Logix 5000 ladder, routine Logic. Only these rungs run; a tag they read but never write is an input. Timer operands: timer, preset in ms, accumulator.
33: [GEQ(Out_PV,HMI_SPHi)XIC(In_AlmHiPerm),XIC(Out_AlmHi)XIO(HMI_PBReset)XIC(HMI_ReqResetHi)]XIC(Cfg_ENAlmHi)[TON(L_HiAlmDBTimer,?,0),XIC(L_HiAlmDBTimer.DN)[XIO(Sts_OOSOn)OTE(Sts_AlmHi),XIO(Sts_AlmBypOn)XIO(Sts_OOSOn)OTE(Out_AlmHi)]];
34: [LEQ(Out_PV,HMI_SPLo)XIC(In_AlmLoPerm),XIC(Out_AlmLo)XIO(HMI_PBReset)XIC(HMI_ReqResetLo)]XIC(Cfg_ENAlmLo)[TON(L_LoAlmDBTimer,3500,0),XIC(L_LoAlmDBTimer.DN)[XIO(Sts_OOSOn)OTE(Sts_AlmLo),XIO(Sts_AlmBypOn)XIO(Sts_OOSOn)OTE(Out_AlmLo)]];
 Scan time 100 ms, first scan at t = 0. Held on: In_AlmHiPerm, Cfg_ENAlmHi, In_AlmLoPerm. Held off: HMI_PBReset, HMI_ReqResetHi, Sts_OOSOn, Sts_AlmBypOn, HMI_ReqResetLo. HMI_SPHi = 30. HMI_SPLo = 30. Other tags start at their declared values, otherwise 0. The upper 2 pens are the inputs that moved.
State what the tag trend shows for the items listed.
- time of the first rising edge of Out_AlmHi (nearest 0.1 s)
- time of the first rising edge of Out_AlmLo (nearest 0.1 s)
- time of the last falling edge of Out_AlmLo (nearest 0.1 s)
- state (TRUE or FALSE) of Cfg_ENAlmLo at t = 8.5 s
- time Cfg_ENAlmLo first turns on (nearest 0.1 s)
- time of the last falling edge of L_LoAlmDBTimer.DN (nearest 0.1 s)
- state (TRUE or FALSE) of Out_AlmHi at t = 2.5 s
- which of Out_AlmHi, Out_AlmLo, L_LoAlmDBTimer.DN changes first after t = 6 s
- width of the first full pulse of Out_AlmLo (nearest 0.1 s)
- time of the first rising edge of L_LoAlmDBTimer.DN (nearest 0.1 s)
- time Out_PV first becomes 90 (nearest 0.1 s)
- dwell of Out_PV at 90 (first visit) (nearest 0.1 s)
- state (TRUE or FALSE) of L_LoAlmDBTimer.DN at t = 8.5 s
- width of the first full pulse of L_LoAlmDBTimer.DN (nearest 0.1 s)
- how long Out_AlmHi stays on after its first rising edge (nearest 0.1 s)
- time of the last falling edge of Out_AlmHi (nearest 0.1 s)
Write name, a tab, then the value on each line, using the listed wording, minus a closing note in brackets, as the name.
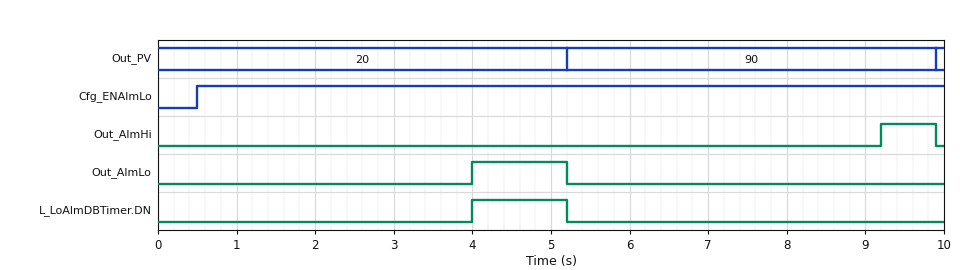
time of the first rising edge of Out_AlmHi	9.2 s
time of the first rising edge of Out_AlmLo	4.0 s
time of the last falling edge of Out_AlmLo	5.2 s
state (TRUE or FALSE) of Cfg_ENAlmLo at t = 8.5 s	TRUE
time Cfg_ENAlmLo first turns on	0.5 s
time of the last falling edge of L_LoAlmDBTimer.DN	5.2 s
state (TRUE or FALSE) of Out_AlmHi at t = 2.5 s	FALSE
which of Out_AlmHi, Out_AlmLo, L_LoAlmDBTimer.DN changes first after t = 6 s	Out_AlmHi
width of the first full pulse of Out_AlmLo	1.2 s
time of the first rising edge of L_LoAlmDBTimer.DN	4.0 s
time Out_PV first becomes 90	5.2 s
dwell of Out_PV at 90 (first visit)	4.7 s
state (TRUE or FALSE) of L_LoAlmDBTimer.DN at t = 8.5 s	FALSE
width of the first full pulse of L_LoAlmDBTimer.DN	1.2 s
how long Out_AlmHi stays on after its first rising edge	0.7 s
time of the last falling edge of Out_AlmHi	9.9 s
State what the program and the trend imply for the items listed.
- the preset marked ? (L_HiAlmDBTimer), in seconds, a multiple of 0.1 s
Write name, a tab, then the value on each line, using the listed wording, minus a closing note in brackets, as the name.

the preset marked ? (L_HiAlmDBTimer), in seconds, a multiple of 0.1 s	4.0 s
